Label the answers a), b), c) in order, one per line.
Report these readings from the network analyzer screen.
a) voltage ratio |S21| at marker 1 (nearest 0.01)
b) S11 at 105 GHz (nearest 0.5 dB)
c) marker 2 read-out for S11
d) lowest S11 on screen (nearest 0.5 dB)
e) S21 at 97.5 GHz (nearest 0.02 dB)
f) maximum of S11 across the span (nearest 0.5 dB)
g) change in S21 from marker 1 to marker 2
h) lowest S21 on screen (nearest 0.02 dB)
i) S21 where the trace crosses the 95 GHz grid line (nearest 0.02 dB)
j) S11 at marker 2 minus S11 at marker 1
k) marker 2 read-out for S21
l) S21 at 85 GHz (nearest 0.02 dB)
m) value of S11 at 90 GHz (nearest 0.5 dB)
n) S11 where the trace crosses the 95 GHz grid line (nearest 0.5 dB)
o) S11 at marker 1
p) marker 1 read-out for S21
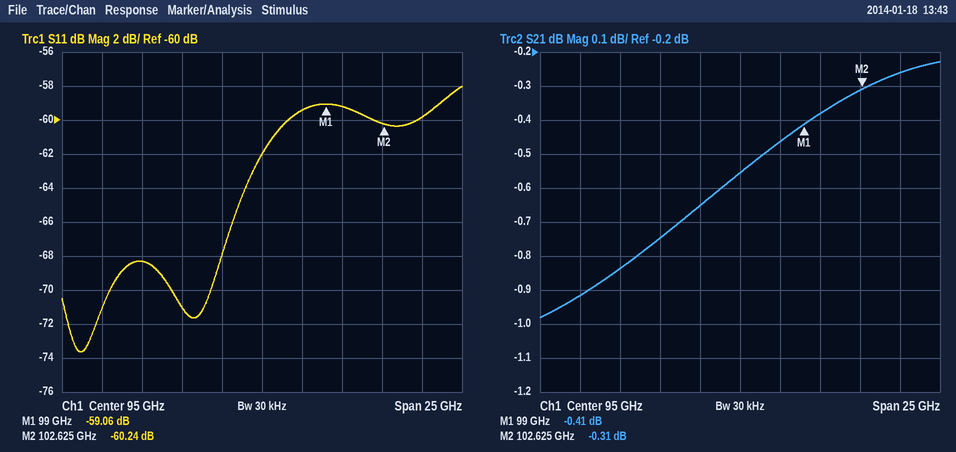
a) 0.95
b) -60.0 dB
c) -60.24 dB
d) -73.5 dB
e) -0.46 dB
f) -58.0 dB
g) 0.10 dB
h) -0.98 dB
i) -0.56 dB
j) -1.18 dB
k) -0.31 dB
l) -0.92 dB
m) -71.0 dB
n) -62.0 dB
o) -59.06 dB
p) -0.41 dB
